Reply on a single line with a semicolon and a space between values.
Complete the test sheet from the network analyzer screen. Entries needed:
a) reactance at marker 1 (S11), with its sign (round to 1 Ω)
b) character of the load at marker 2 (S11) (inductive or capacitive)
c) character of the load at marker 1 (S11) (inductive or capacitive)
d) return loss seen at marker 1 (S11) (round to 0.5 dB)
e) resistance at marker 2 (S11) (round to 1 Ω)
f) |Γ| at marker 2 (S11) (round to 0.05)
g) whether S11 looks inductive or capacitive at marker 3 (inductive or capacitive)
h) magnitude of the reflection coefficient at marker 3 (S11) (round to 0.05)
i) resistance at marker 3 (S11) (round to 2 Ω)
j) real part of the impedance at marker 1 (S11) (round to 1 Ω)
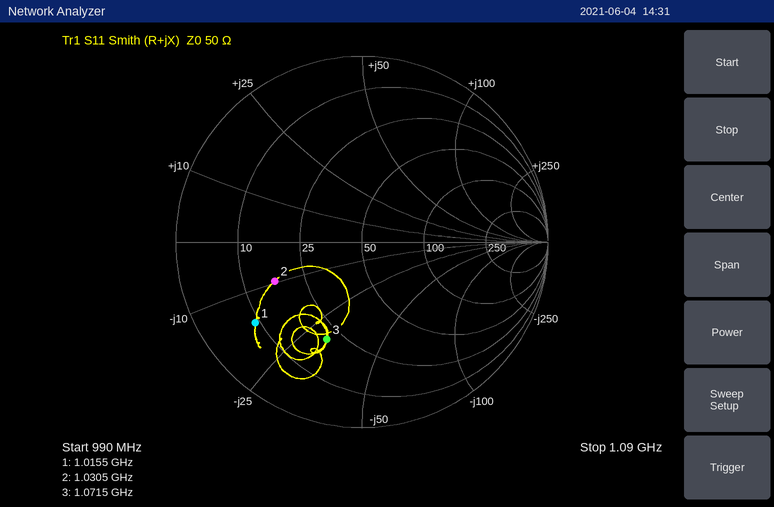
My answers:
-16 Ω; capacitive; capacitive; 3.0 dB; 17 Ω; 0.50; capacitive; 0.55; 20 Ω; 9 Ω
